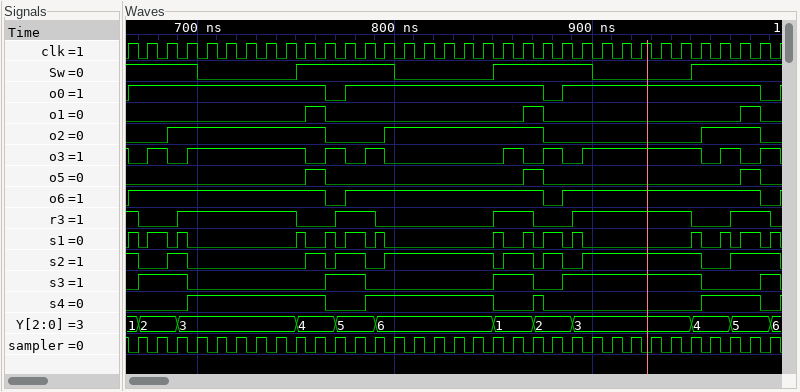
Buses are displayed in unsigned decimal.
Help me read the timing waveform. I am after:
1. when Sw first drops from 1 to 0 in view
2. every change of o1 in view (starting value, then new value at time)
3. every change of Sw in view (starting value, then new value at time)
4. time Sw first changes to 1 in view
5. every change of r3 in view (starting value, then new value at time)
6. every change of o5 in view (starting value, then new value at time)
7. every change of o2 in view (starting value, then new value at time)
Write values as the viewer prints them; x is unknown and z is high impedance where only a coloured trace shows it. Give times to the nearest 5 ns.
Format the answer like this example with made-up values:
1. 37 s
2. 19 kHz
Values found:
1. 700 ns
2. 0, 1 at 755 ns, 0 at 765 ns, 1 at 865 ns, 0 at 875 ns, 1 at 975 ns, 0 at 985 ns
3. 1, 0 at 700 ns, 1 at 750 ns, 0 at 800 ns, 1 at 850 ns, 0 at 900 ns, 1 at 950 ns
4. 750 ns
5. 1, 0 at 670 ns, 1 at 690 ns, 0 at 750 ns, 1 at 770 ns, 0 at 790 ns, 1 at 850 ns, 0 at 870 ns, 1 at 890 ns, 0 at 950 ns, 1 at 970 ns, 0 at 990 ns
6. 0, 1 at 755 ns, 0 at 765 ns, 1 at 865 ns, 0 at 875 ns, 1 at 975 ns, 0 at 985 ns
7. 0, 1 at 685 ns, 0 at 765 ns, 1 at 795 ns, 0 at 875 ns, 1 at 955 ns, 0 at 985 ns
